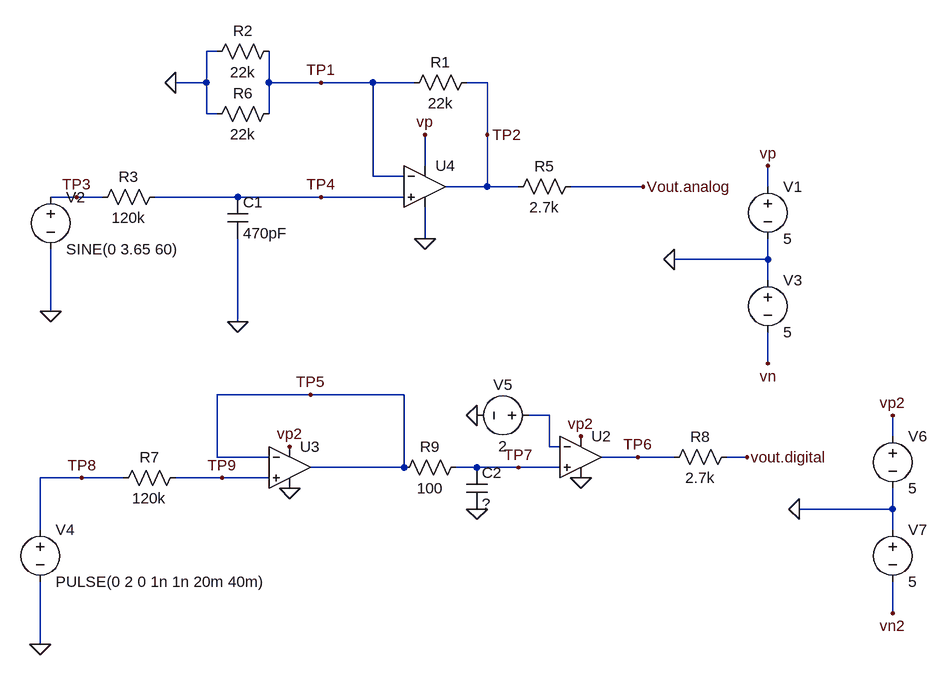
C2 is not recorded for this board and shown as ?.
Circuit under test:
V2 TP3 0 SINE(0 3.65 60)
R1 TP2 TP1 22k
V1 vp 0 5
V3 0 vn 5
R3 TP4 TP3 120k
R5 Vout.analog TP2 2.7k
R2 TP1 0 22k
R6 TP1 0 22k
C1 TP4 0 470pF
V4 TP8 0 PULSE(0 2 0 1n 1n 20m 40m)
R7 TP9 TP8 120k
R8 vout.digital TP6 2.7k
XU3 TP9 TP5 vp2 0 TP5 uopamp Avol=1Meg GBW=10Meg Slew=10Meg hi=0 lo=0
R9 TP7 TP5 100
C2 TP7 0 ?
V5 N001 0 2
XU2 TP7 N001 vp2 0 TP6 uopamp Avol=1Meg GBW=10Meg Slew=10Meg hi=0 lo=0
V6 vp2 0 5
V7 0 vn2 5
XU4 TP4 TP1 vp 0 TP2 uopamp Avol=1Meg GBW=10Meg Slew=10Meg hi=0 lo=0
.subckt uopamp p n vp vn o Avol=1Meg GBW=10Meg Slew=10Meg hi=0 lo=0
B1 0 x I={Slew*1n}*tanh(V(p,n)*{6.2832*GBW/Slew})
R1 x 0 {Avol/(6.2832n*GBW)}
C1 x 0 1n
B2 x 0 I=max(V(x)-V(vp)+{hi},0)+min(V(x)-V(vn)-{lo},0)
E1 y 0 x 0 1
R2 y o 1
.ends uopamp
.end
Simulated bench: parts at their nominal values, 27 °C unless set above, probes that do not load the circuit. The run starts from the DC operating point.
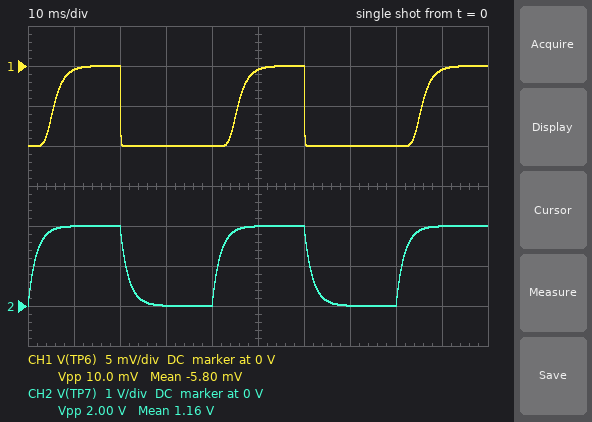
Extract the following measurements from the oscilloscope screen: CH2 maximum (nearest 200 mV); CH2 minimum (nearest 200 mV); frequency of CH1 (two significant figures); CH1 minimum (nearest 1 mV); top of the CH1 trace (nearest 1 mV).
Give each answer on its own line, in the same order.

2.0 V
0 V
25 Hz
-10 mV
0 V
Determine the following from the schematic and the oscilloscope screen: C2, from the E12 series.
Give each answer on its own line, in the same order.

18 µF
